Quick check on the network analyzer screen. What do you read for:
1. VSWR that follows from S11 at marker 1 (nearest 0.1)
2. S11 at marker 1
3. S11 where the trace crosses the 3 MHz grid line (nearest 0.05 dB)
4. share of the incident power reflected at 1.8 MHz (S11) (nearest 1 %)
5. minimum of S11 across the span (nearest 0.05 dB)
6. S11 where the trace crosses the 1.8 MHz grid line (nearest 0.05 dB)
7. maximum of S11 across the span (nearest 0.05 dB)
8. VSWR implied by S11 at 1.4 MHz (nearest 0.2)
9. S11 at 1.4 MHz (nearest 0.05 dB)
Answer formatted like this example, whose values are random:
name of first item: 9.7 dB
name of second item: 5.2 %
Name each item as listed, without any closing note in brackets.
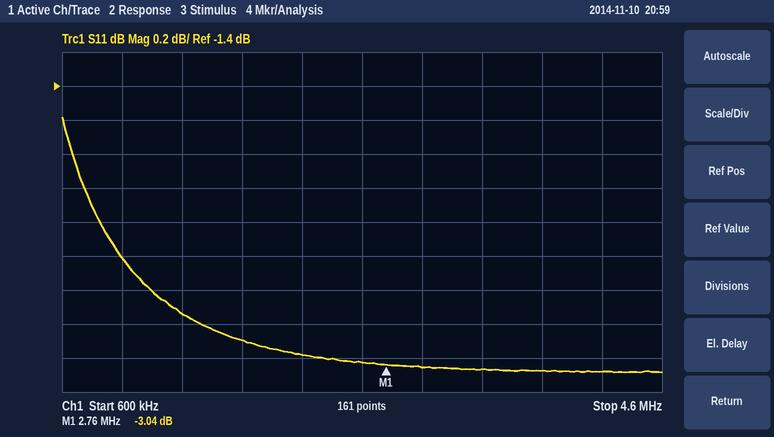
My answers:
VSWR that follows from S11 at marker 1: 5.8
S11 at marker 1: -3.04 dB
S11 where the trace crosses the 3 MHz grid line: -3.05 dB
share of the incident power reflected at 1.8 MHz (S11): 51 %
minimum of S11 across the span: -3.10 dB
S11 where the trace crosses the 1.8 MHz grid line: -2.90 dB
maximum of S11 across the span: -1.60 dB
VSWR implied by S11 at 1.4 MHz: 6.4
S11 at 1.4 MHz: -2.75 dB
